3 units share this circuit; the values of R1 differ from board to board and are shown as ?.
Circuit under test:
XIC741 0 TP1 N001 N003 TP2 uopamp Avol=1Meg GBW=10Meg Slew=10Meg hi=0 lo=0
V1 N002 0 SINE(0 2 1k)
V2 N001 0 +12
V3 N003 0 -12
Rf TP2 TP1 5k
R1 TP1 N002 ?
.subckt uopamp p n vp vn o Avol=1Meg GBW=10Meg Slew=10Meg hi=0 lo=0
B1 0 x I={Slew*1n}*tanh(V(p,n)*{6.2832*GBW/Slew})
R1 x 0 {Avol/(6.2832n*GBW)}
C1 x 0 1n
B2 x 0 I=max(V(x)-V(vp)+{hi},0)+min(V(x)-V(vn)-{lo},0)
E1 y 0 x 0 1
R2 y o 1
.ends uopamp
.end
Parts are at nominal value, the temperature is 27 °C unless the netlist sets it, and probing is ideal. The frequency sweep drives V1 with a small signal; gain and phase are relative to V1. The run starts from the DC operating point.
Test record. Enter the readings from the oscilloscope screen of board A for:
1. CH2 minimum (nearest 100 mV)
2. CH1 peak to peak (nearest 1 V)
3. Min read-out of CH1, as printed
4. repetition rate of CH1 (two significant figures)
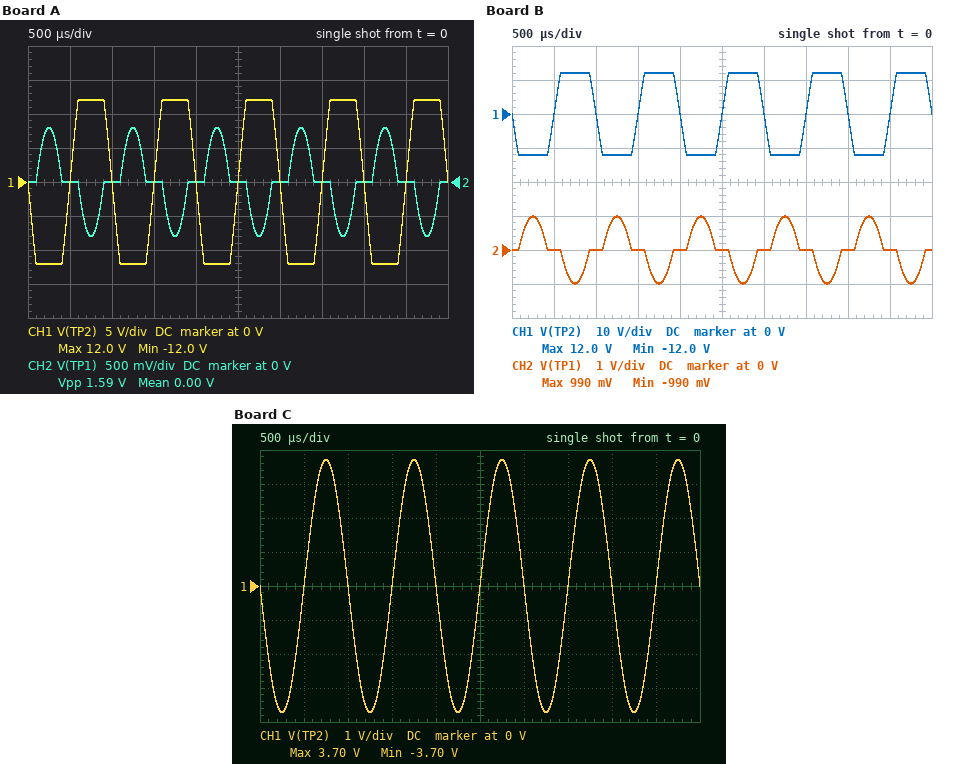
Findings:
-800 mV
24 V
-12.0 V
1.0 kHz
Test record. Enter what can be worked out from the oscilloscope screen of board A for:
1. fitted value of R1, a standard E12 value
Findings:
470 Ω
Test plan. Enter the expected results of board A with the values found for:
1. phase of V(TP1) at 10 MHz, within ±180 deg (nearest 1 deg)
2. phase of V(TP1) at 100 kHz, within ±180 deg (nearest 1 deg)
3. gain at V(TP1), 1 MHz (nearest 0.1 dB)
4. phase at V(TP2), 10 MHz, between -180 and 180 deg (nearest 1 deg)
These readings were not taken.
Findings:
5 deg
83 deg
-3.2 dB
95 deg
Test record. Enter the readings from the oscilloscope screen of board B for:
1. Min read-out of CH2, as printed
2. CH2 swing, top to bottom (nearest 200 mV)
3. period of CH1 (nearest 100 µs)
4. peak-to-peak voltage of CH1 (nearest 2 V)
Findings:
-990 mV
2.0 V
1.0 ms
24 V
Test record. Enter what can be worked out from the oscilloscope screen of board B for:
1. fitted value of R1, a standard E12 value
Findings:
390 Ω
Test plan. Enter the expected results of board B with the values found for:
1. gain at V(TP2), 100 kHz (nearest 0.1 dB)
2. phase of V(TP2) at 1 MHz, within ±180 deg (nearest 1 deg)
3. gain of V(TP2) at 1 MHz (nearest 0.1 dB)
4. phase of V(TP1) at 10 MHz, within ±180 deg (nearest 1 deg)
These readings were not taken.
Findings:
22.1 dB
126 deg
17.5 dB
4 deg
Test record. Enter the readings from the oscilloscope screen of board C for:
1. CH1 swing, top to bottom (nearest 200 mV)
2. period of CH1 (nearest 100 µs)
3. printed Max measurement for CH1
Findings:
7.4 V
1.0 ms
3.70 V
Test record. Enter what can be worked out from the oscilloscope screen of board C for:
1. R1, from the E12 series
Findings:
2.7 kΩ
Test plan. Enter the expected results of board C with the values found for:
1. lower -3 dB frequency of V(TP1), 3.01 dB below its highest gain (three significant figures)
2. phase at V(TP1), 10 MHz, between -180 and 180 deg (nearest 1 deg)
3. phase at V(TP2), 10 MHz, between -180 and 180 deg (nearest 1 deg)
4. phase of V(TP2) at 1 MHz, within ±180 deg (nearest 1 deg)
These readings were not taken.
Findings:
3.51 MHz
19 deg
109 deg
164 deg
